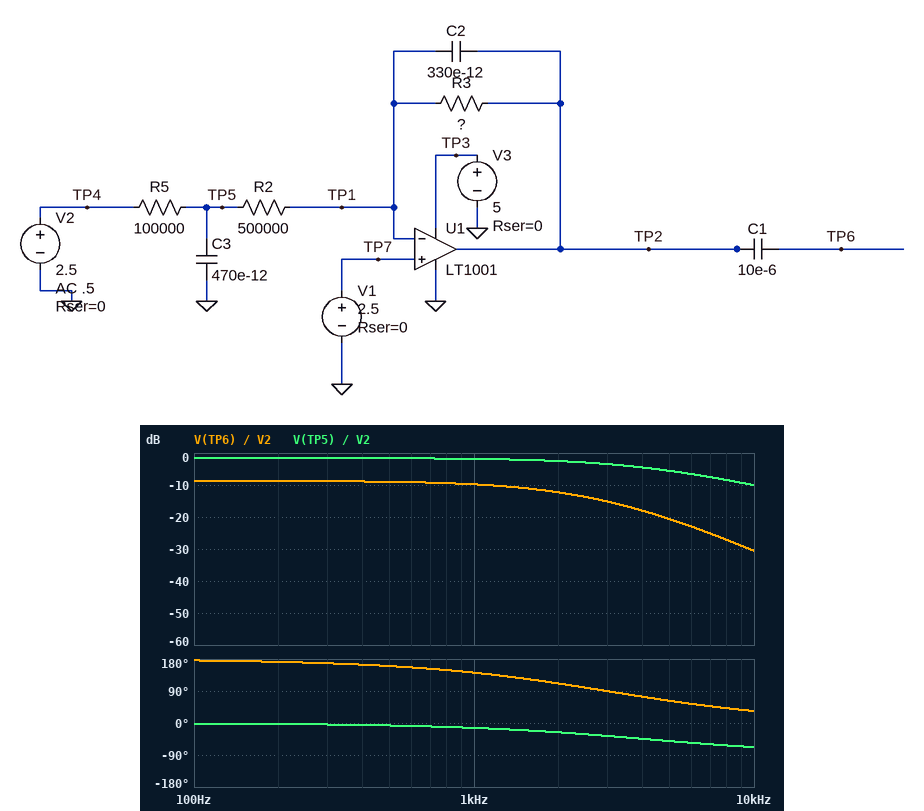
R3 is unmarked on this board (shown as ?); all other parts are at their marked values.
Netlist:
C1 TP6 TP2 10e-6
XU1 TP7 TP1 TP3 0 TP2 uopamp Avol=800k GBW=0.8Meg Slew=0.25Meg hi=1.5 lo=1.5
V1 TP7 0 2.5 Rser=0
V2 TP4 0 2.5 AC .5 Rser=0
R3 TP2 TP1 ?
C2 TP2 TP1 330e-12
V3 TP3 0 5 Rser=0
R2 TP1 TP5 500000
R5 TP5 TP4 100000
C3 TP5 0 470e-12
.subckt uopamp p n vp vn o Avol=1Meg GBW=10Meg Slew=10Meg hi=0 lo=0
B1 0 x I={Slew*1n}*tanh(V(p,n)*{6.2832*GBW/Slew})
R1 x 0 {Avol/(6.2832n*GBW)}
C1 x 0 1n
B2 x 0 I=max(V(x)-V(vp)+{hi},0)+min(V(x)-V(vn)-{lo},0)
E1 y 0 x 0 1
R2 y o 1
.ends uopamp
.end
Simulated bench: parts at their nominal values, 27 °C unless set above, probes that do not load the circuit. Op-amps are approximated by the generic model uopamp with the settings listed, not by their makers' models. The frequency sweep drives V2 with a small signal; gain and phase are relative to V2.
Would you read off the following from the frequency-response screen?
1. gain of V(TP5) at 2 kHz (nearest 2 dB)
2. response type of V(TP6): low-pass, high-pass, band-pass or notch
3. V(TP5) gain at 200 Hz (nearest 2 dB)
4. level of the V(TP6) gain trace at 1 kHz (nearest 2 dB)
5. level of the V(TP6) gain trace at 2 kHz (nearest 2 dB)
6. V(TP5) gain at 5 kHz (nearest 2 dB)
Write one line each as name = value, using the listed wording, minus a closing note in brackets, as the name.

gain of V(TP5) at 2 kHz = -2 dB
response type of V(TP6): low-pass, high-pass, band-pass or notch = low-pass
V(TP5) gain at 200 Hz = -2 dB
level of the V(TP6) gain trace at 1 kHz = -10 dB
level of the V(TP6) gain trace at 2 kHz = -12 dB
V(TP5) gain at 5 kHz = -6 dB
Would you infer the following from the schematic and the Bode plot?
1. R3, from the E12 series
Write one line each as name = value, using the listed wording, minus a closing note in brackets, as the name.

R3, from the E12 series = 220 kΩ
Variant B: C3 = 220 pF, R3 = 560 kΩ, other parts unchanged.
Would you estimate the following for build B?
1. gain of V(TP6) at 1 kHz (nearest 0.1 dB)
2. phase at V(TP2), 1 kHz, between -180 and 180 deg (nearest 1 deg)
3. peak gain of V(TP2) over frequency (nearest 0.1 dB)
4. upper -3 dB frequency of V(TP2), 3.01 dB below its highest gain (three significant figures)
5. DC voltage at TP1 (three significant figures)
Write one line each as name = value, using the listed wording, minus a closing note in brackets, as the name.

gain of V(TP6) at 1 kHz = -4.4 dB
phase at V(TP2), 1 kHz, between -180 and 180 deg = 124 deg
peak gain of V(TP2) over frequency = -0.6 dB
upper -3 dB frequency of V(TP2), 3.01 dB below its highest gain = 852 Hz
DC voltage at TP1 = 2.50 V
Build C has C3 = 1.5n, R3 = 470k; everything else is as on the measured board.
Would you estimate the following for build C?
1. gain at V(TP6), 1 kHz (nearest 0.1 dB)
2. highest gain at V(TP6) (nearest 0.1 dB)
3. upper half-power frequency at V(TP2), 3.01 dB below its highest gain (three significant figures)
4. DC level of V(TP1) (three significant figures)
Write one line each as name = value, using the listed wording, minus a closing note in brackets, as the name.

gain at V(TP6), 1 kHz = -7.1 dB
highest gain at V(TP6) = -2.1 dB
upper half-power frequency at V(TP2), 3.01 dB below its highest gain = 729 Hz
DC level of V(TP1) = 2.50 V
